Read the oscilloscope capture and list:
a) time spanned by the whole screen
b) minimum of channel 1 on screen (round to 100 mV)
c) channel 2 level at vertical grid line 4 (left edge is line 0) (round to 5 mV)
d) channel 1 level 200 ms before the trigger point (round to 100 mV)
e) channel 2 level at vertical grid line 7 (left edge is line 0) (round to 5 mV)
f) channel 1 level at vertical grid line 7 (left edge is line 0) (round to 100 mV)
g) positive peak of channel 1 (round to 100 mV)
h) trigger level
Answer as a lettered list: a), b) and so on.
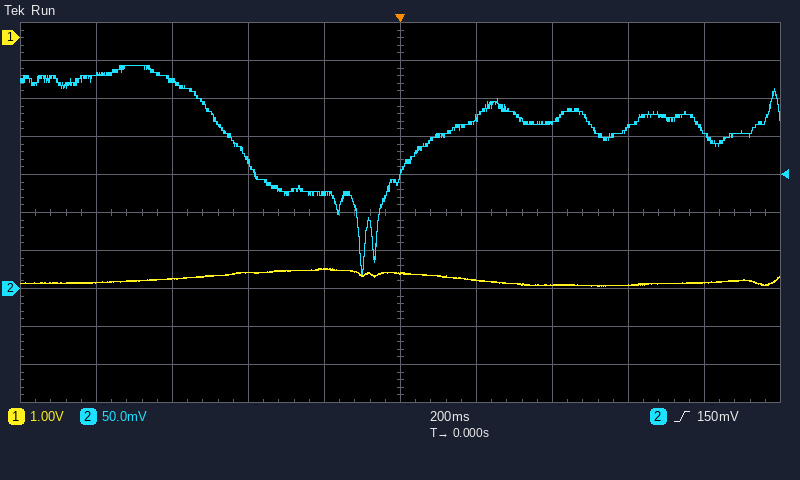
a) 2 s
b) -6.5 V
c) 125 mV
d) -6.1 V
e) 220 mV
f) -6.5 V
g) -6.1 V
h) 150 mV
